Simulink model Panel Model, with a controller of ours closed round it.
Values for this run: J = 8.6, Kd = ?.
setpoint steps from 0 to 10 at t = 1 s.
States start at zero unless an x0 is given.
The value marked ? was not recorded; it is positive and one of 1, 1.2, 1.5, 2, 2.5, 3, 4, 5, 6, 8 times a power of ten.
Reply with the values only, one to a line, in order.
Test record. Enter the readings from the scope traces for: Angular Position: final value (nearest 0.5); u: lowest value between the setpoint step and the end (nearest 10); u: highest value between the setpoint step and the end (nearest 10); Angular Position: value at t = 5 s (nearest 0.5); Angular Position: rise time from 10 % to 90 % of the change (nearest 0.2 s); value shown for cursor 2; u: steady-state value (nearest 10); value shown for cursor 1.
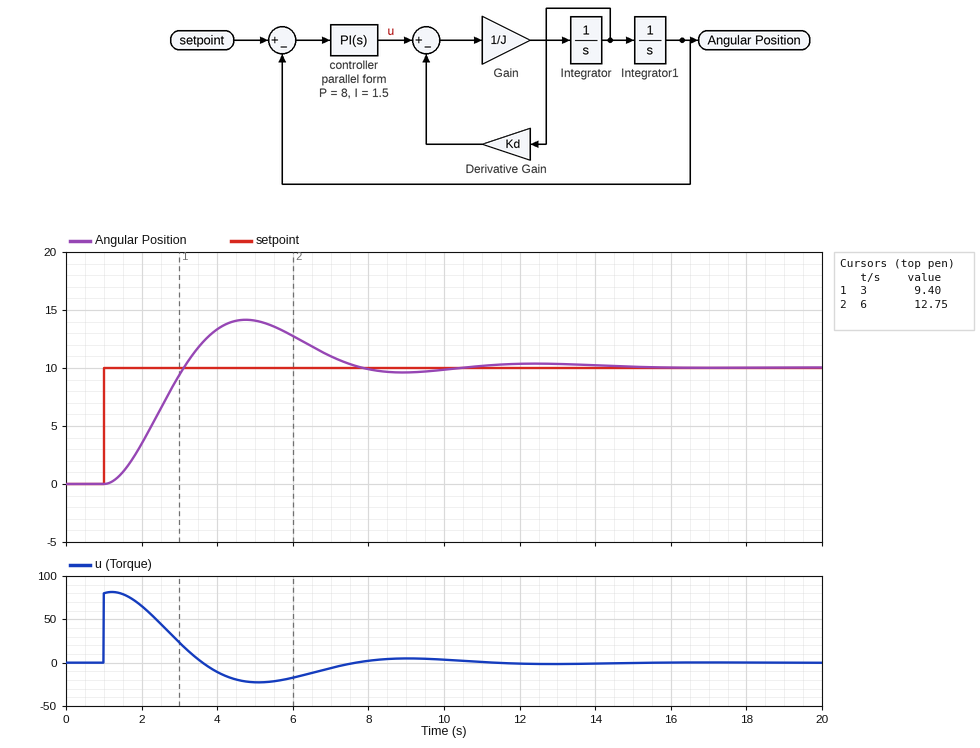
10.0
-20
80
14.0
1.4 s
12.75
0
9.40
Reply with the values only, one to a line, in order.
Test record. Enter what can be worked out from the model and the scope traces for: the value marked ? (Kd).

8
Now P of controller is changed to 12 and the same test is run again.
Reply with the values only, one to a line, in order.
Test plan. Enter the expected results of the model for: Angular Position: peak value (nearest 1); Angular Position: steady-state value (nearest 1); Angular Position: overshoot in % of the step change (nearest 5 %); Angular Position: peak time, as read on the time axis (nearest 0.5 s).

14
10
40 %
4.0 s
